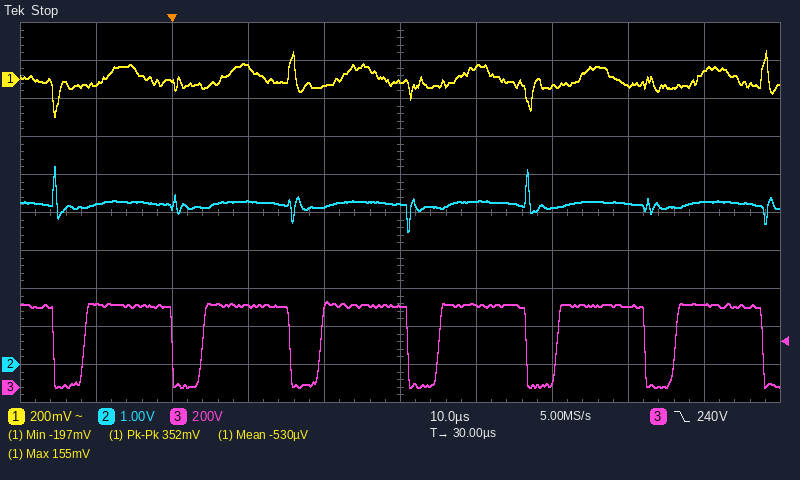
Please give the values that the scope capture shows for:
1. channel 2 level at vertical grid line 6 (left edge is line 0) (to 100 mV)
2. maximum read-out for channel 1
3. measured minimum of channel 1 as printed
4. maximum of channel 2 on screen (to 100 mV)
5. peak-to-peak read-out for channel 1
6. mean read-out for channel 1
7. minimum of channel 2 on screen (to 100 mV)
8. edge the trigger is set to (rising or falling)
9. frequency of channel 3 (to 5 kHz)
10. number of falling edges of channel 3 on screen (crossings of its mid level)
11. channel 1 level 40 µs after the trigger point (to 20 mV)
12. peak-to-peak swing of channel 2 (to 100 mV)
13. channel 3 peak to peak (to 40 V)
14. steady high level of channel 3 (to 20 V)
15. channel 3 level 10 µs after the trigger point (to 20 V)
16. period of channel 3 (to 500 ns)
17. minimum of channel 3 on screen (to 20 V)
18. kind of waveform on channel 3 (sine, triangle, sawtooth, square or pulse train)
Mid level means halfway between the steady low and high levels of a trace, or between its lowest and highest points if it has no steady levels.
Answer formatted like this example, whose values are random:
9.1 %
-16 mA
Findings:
4.3 V
155 mV
-197 mV
5.2 V
352 mV
-530 µV
3.5 V
falling
65 kHz
7
60 mV
1.7 V
440 V
440 V
420 V
15.5 µs
0 V
pulse train
